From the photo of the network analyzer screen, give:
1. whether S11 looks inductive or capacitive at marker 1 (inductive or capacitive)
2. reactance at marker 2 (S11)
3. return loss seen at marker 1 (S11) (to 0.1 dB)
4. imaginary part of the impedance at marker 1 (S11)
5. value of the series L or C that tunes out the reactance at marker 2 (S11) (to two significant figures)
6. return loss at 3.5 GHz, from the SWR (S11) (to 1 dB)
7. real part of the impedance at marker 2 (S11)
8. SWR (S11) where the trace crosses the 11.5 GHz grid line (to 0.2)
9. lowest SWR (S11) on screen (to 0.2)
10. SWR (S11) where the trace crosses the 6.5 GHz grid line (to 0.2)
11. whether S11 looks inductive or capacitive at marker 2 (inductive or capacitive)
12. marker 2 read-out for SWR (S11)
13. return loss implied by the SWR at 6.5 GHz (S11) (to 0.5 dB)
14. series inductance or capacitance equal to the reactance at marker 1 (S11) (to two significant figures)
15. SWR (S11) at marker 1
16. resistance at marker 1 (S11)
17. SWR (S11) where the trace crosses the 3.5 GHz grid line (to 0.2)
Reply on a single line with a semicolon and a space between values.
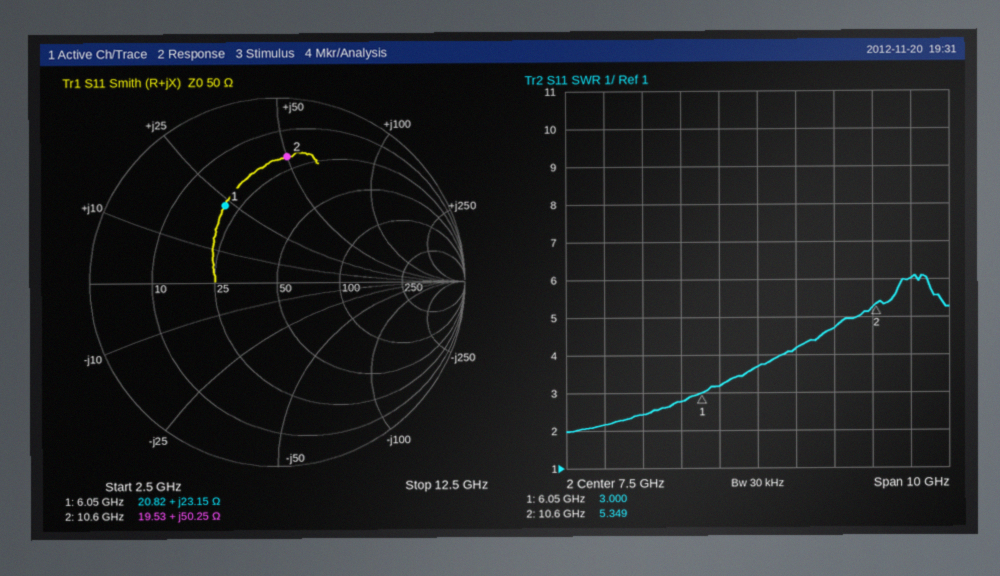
inductive; +50.25 Ω; 6.0 dB; +23.15 Ω; 300 fF; 9 dB; 19.53 Ω; 6.0; 2.0; 3.2; inductive; 5.349; 5.5 dB; 610 pH; 3.000; 20.82 Ω; 2.2
